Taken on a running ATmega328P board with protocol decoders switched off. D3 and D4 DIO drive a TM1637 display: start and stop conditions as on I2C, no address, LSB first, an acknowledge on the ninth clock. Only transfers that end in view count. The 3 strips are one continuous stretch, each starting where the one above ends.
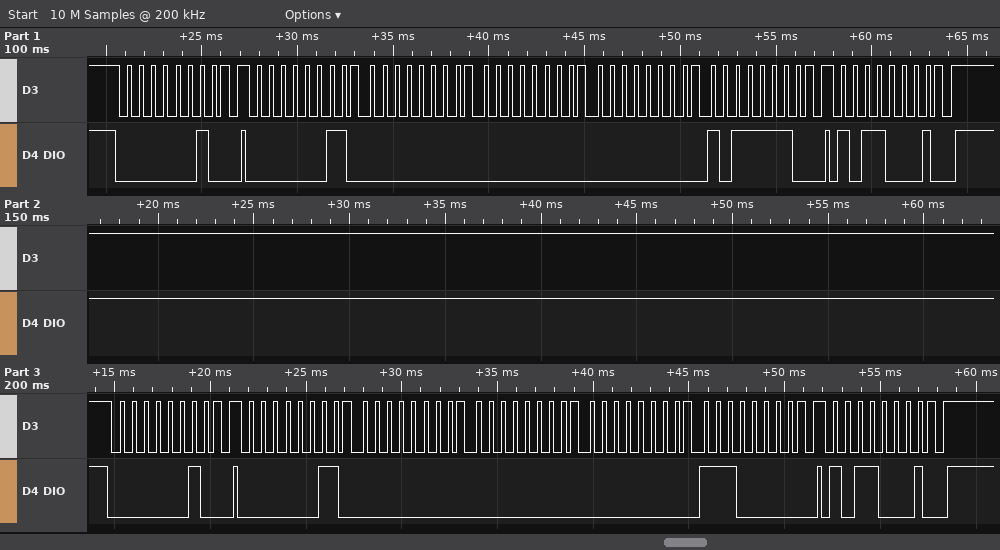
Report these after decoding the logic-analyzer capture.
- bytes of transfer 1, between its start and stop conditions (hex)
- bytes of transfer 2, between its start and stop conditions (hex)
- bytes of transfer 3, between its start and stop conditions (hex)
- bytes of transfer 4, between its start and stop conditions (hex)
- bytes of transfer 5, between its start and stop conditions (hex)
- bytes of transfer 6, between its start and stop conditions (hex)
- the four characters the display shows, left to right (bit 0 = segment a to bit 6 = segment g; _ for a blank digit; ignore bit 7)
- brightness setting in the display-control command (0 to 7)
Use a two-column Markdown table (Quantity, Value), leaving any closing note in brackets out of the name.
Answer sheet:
| Quantity | Value |
|---|---|
| bytes of transfer 1, between its start and stop conditions | 40 |
| bytes of transfer 2, between its start and stop conditions | C0 00 00 00 7D |
| bytes of transfer 3, between its start and stop conditions | 8D |
| bytes of transfer 4, between its start and stop conditions | 40 |
| bytes of transfer 5, between its start and stop conditions | C0 00 00 00 07 |
| bytes of transfer 6, between its start and stop conditions | 8D |
| the four characters the display shows, left to right | ___7 |
| brightness setting in the display-control command | 5 |
